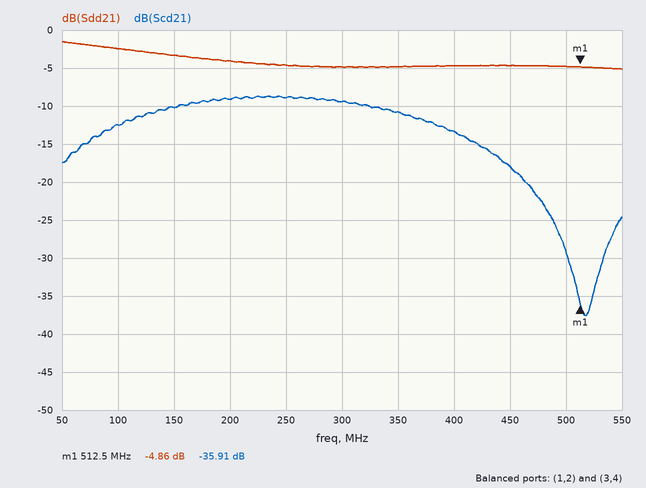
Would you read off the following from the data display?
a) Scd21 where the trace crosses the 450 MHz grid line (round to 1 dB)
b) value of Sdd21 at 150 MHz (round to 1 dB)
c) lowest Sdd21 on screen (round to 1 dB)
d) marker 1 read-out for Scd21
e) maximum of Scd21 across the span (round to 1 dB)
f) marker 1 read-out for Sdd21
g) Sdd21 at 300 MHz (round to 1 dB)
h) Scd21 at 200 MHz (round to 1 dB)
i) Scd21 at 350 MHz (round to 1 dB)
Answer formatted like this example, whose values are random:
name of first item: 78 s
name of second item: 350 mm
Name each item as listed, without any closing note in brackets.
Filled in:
Scd21 where the trace crosses the 450 MHz grid line: -18 dB
value of Sdd21 at 150 MHz: -3 dB
lowest Sdd21 on screen: -5 dB
marker 1 read-out for Scd21: -35.91 dB
maximum of Scd21 across the span: -9 dB
marker 1 read-out for Sdd21: -4.86 dB
Sdd21 at 300 MHz: -5 dB
Scd21 at 200 MHz: -9 dB
Scd21 at 350 MHz: -11 dB
